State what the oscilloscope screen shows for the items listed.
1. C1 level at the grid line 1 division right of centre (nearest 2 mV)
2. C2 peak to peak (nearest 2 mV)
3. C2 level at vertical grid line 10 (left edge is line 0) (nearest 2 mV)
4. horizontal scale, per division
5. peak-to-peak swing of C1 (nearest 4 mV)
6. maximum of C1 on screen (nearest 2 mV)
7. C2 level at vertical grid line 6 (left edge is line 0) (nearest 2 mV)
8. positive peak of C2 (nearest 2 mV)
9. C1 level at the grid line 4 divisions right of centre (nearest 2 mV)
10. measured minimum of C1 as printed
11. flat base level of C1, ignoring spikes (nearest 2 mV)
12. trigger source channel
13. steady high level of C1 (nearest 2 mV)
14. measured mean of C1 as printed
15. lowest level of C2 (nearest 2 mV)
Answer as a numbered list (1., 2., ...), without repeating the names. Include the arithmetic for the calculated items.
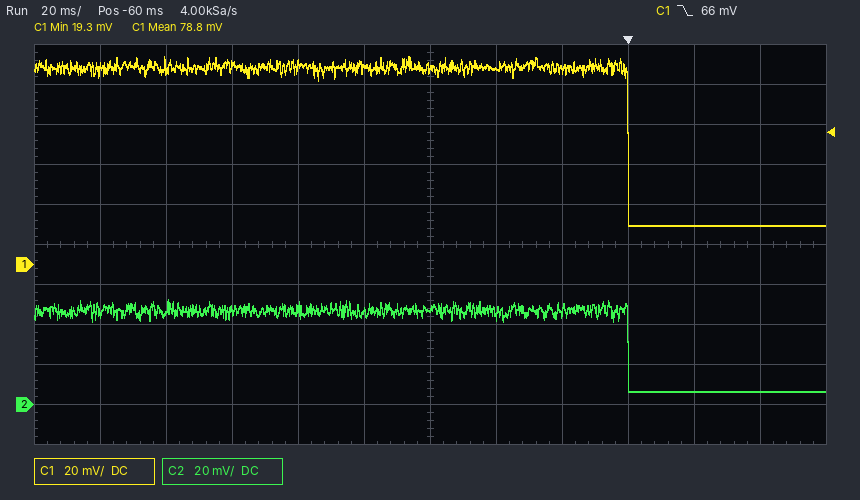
1. 98 mV
2. 52 mV − (6 mV) = 46 mV
3. 6 mV
4. 20 ms
5. 84 mV
6. 104 mV
7. 48 mV
8. 52 mV
9. 20 mV
10. 19.3 mV
11. 20 mV
12. C1
13. 98 mV
14. 78.8 mV
15. 6 mV
